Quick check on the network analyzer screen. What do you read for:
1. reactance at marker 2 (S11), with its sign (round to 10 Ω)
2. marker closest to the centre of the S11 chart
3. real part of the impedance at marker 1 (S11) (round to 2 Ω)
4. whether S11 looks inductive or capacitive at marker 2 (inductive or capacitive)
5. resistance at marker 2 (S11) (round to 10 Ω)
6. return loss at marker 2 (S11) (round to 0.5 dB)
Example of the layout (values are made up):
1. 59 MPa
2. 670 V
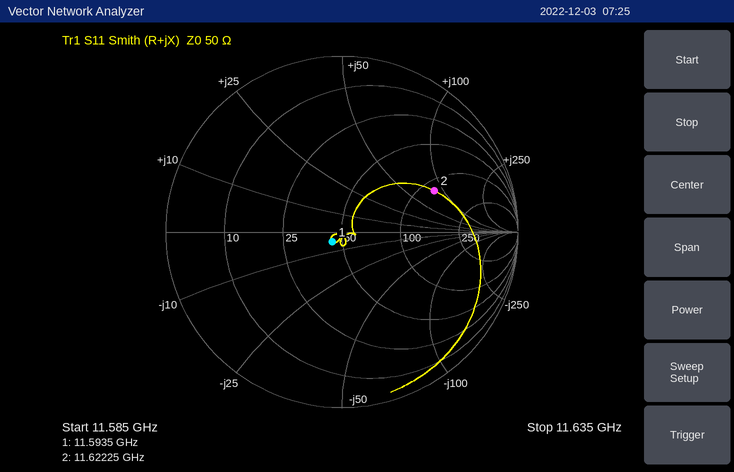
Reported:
1. +80 Ω
2. marker 1
3. 44 Ω
4. inductive
5. 120 Ω
6. 5.0 dB
